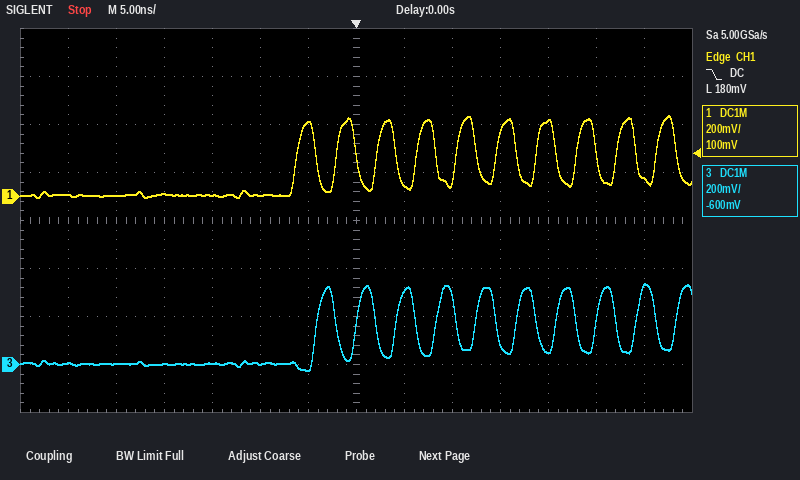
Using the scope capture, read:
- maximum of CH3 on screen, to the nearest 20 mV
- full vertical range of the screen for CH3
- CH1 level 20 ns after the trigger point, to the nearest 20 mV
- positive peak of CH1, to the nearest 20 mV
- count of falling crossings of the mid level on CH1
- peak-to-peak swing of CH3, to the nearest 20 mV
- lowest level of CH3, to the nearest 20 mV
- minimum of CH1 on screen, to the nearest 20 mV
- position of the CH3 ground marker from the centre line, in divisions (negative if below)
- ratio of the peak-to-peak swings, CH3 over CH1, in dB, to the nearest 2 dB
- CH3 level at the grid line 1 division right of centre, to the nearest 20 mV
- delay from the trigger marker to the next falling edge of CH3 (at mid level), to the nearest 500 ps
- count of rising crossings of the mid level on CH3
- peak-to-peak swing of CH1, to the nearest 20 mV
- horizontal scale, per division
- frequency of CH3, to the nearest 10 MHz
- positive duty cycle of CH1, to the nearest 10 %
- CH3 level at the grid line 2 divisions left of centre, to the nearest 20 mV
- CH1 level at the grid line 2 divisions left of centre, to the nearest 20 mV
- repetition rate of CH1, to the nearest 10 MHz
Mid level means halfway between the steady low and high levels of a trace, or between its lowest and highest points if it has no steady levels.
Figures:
340 mV
1.6 V
320 mV
340 mV
10
360 mV
-20 mV
0 mV
-3.0 div
0 dB
300 mV
2.0 ns
10
340 mV
5 ns
240 MHz
50 %
0 mV
0 mV
240 MHz
